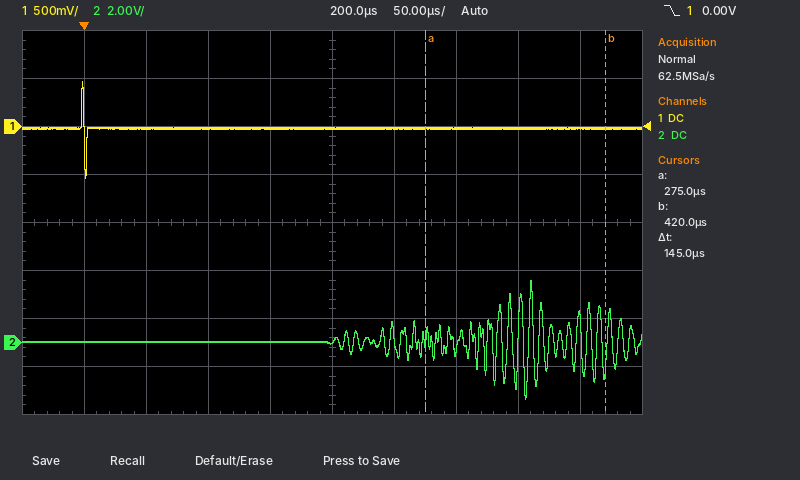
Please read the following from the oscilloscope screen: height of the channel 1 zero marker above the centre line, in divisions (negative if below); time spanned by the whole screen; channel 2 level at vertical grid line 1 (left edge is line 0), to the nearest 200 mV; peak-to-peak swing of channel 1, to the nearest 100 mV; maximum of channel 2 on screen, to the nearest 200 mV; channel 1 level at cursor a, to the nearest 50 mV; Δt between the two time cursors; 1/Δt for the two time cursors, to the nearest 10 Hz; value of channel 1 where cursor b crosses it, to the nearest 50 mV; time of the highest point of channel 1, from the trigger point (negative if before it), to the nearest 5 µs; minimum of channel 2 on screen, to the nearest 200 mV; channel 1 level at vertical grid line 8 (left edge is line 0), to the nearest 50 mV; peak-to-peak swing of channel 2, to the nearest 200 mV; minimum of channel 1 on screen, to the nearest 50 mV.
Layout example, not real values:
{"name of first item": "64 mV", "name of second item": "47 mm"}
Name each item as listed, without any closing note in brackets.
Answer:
{"height of the channel 1 zero marker above the centre line, in divisions": "+2.0 div", "time spanned by the whole screen": "500 µs", "channel 2 level at vertical grid line 1 (left edge is line 0), to the nearest 200 mV": "0.0 V", "peak-to-peak swing of channel 1, to the nearest 100 mV": "1.00 V", "maximum of channel 2 on screen, to the nearest 200 mV": "2.6 V", "channel 1 level at cursor a, to the nearest 50 mV": "0 mV", "Δt between the two time cursors": "145 µs", "1/Δt for the two time cursors, to the nearest 10 Hz": "6.90 kHz", "value of channel 1 where cursor b crosses it, to the nearest 50 mV": "0 mV", "time of the highest point of channel 1, from the trigger point (negative if before it), to the nearest 5 µs": "0 µs", "minimum of channel 2 on screen, to the nearest 200 mV": "-2.4 V", "channel 1 level at vertical grid line 8 (left edge is line 0), to the nearest 50 mV": "0 mV", "peak-to-peak swing of channel 2, to the nearest 200 mV": "5.0 V", "minimum of channel 1 on screen, to the nearest 50 mV": "-550 mV"}
